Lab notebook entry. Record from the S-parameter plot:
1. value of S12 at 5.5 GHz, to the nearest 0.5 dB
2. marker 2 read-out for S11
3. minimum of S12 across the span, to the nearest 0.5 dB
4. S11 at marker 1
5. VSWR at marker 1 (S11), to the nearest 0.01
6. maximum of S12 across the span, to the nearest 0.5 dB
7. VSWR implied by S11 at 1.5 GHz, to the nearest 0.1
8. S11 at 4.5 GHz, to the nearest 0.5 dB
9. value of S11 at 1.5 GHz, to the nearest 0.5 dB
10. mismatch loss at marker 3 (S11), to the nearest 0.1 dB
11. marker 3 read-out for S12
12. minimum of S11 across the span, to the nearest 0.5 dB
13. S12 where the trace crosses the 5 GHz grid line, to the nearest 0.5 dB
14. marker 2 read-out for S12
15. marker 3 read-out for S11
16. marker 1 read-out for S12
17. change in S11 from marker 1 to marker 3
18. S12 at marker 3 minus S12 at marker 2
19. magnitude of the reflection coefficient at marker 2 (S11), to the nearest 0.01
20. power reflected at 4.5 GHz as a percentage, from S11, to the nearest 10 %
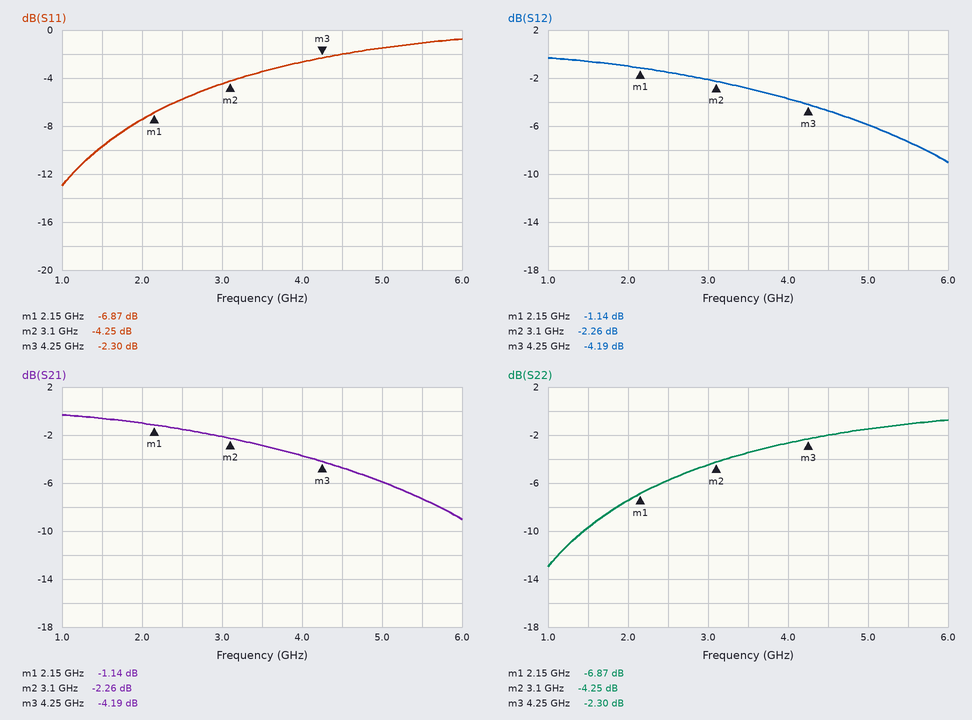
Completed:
-7.5 dB
-4.25 dB
-9.0 dB
-6.87 dB
2.66
-0.5 dB
2.0
-2.0 dB
-9.5 dB
3.9 dB
-4.19 dB
-13.0 dB
-6.0 dB
-2.26 dB
-2.30 dB
-1.14 dB
4.57 dB
-1.93 dB
0.61
60 %
